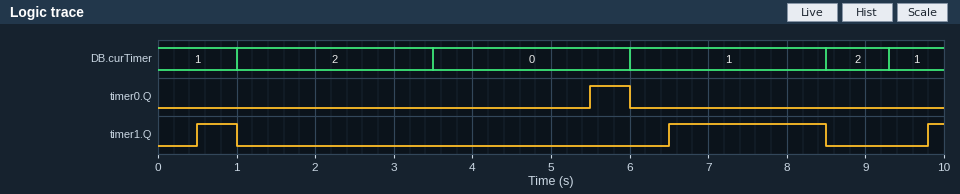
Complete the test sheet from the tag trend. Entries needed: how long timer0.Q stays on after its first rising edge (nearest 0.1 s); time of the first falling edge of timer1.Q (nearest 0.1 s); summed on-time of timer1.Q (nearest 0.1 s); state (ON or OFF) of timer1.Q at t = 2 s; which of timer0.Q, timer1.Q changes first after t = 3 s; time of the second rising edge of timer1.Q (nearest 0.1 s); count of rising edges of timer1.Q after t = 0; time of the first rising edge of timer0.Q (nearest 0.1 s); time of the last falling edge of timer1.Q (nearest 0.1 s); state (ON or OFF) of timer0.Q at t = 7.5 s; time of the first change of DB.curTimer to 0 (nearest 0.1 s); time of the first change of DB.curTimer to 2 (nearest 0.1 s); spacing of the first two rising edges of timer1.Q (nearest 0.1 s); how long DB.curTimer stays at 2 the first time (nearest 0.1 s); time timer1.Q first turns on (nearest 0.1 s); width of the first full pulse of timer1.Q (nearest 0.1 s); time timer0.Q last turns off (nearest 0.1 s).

0.5 s
1.0 s
2.7 s
OFF
timer0.Q
6.5 s
3
5.5 s
8.5 s
OFF
3.5 s
1.0 s
6.0 s
2.5 s
0.5 s
0.5 s
6.0 s
